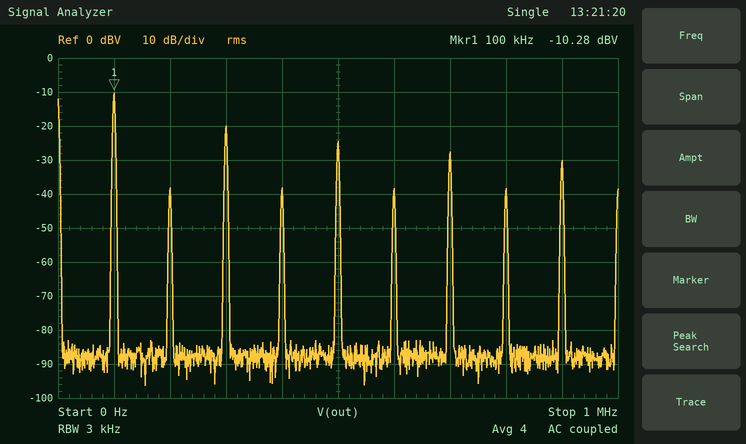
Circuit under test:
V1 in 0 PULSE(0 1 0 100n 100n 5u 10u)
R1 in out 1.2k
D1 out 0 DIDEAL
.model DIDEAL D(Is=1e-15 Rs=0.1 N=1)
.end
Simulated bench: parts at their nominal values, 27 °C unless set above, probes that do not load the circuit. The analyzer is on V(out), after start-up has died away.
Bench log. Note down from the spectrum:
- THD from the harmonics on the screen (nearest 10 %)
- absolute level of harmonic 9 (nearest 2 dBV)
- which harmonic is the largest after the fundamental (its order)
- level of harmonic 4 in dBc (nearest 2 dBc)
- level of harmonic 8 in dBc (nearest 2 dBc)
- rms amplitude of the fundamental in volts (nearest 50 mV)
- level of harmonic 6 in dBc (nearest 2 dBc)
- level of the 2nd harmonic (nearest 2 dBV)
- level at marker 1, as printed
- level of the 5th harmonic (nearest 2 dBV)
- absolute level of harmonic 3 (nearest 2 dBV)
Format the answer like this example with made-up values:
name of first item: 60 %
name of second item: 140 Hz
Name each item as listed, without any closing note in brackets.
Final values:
THD from the harmonics on the screen: 40 %
absolute level of harmonic 9: -30 dBV
which harmonic is the largest after the fundamental: 3
level of harmonic 4 in dBc: -28 dBc
level of harmonic 8 in dBc: -28 dBc
rms amplitude of the fundamental in volts: 300 mV
level of harmonic 6 in dBc: -28 dBc
level of the 2nd harmonic: -38 dBV
level at marker 1, as printed: -10.28 dBV
level of the 5th harmonic: -24 dBV
absolute level of harmonic 3: -20 dBV
